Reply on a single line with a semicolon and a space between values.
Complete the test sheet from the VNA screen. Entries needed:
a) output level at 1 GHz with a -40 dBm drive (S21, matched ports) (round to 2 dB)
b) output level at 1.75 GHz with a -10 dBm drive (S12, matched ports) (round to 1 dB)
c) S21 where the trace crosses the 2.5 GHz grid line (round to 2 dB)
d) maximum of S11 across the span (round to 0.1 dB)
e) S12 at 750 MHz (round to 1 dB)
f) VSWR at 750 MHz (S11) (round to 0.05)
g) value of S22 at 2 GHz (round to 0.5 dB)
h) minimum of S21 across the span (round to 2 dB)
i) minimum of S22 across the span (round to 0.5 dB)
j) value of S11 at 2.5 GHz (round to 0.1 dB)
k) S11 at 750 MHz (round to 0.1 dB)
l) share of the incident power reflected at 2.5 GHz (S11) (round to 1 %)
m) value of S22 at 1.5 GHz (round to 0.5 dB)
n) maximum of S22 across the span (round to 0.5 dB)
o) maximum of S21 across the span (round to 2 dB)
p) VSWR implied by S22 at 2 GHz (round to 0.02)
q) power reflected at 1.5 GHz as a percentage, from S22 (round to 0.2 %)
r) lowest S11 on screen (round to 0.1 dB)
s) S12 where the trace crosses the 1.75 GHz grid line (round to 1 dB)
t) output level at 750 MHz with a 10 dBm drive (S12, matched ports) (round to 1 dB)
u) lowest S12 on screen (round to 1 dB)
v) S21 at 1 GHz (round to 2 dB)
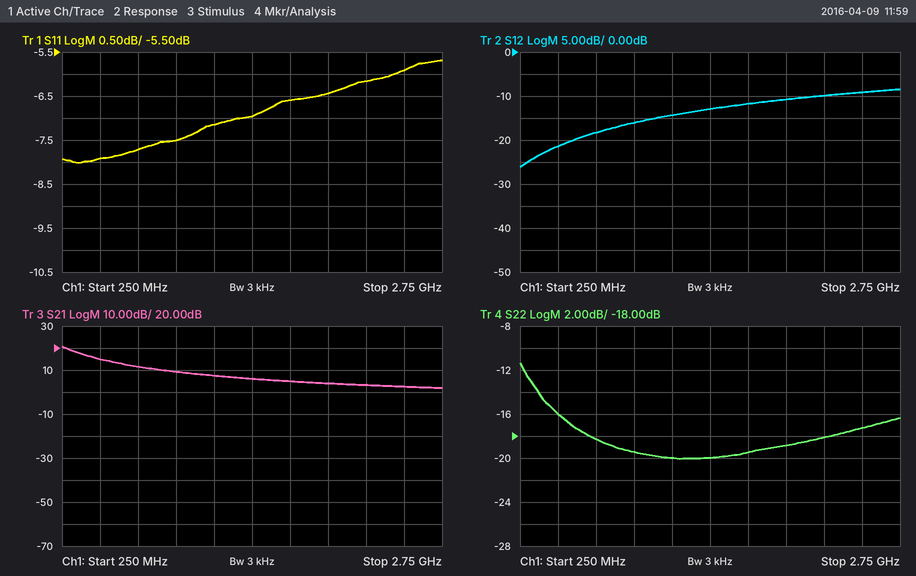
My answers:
-30 dBm; -22 dBm; 2 dB; -5.7 dB; -18 dB; 2.40; -19.0 dB; 2 dB; -20.0 dB; -5.9 dB; -7.7 dB; 26 %; -20.0 dB; -11.5 dB; 20 dB; 1.26; 1.0 %; -8.0 dB; -12 dB; -8 dBm; -26 dB; 10 dB
